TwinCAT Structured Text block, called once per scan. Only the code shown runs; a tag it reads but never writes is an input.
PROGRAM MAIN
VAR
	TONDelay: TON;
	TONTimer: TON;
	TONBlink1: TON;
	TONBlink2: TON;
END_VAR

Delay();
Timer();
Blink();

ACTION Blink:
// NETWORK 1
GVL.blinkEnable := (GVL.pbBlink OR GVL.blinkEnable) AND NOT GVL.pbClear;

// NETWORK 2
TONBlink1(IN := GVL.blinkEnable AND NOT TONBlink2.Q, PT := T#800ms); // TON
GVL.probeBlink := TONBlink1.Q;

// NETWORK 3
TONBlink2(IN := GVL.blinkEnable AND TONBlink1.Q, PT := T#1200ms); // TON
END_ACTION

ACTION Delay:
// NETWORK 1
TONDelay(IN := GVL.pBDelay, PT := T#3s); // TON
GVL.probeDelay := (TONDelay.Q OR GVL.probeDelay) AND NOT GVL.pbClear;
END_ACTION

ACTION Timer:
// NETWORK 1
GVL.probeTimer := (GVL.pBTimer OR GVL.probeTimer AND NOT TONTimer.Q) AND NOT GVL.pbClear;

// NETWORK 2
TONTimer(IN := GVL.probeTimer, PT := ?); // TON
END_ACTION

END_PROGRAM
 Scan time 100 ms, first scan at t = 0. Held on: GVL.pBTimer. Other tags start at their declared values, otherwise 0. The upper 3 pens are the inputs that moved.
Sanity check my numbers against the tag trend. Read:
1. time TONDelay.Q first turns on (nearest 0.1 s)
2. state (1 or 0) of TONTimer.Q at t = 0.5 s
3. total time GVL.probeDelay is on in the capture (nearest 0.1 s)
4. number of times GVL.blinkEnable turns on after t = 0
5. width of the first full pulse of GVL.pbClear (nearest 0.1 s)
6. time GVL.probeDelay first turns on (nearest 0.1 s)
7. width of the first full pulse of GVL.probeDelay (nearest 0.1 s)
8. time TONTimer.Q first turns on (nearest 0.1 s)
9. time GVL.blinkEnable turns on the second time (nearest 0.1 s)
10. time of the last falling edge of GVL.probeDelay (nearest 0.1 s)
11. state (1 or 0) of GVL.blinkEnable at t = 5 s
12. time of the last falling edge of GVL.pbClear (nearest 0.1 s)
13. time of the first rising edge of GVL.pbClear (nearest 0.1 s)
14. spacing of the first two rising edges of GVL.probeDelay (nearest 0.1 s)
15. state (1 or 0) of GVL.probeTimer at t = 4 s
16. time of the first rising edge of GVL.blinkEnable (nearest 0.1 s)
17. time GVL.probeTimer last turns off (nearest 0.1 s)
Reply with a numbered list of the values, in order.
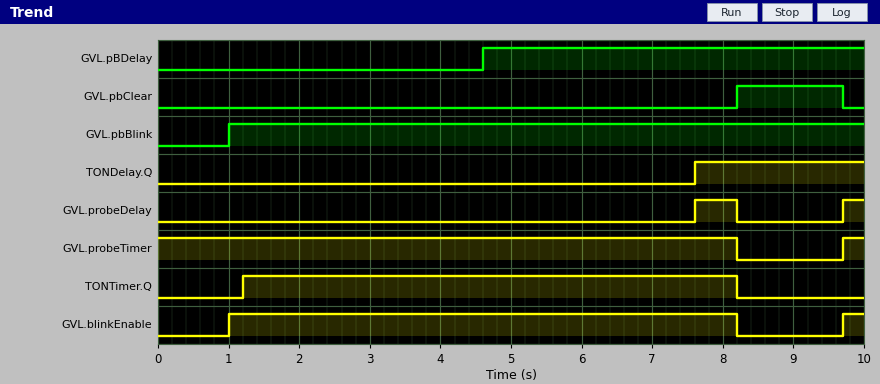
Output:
1. 7.6 s
2. 0
3. 0.9 s
4. 2
5. 1.5 s
6. 7.6 s
7. 0.6 s
8. 1.2 s
9. 9.7 s
10. 8.2 s
11. 1
12. 9.7 s
13. 8.2 s
14. 2.1 s
15. 1
16. 1.0 s
17. 8.2 s
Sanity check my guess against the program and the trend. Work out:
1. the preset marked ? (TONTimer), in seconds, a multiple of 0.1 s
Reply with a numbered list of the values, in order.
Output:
1. 1.2 s
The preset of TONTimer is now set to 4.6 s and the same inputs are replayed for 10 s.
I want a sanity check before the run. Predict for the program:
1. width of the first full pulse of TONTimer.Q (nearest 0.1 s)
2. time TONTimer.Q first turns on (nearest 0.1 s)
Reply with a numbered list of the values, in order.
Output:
1. 3.6 s
2. 4.6 s
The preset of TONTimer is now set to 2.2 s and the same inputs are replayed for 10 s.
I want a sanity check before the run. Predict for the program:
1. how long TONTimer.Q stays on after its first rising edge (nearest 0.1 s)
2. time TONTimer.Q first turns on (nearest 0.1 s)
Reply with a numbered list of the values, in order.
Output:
1. 6.0 s
2. 2.2 s
